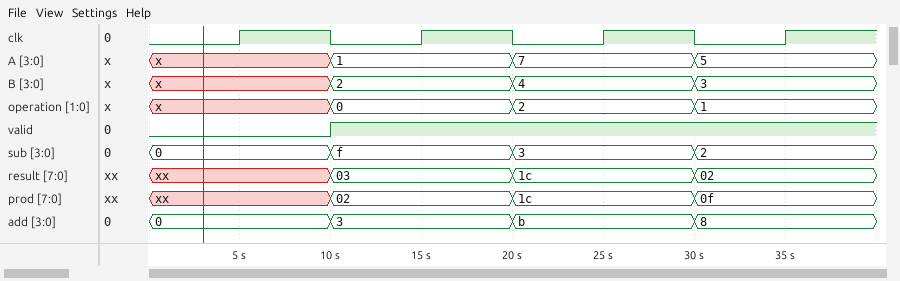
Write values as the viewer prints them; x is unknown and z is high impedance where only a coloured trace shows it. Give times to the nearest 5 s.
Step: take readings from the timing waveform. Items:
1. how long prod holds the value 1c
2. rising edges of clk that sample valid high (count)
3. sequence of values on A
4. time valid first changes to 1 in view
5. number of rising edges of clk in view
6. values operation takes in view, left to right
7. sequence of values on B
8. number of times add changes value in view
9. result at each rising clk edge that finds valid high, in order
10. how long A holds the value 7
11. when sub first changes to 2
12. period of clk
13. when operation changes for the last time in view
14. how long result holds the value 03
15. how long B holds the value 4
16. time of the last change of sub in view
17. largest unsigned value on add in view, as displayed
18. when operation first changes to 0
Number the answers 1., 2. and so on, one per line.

1. 10 s
2. 3
3. x, 1, 7, 5
4. 10 s
5. 4
6. x, 0, 2, 1
7. x, 2, 4, 3
8. 3
9. 03, 1c, 02
10. 10 s
11. 30 s
12. 10 s
13. 30 s
14. 10 s
15. 10 s
16. 30 s
17. b
18. 10 s
